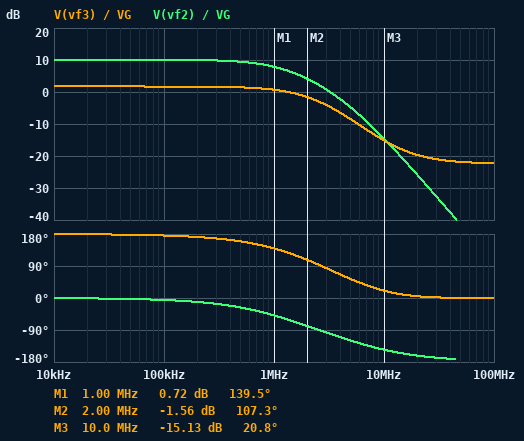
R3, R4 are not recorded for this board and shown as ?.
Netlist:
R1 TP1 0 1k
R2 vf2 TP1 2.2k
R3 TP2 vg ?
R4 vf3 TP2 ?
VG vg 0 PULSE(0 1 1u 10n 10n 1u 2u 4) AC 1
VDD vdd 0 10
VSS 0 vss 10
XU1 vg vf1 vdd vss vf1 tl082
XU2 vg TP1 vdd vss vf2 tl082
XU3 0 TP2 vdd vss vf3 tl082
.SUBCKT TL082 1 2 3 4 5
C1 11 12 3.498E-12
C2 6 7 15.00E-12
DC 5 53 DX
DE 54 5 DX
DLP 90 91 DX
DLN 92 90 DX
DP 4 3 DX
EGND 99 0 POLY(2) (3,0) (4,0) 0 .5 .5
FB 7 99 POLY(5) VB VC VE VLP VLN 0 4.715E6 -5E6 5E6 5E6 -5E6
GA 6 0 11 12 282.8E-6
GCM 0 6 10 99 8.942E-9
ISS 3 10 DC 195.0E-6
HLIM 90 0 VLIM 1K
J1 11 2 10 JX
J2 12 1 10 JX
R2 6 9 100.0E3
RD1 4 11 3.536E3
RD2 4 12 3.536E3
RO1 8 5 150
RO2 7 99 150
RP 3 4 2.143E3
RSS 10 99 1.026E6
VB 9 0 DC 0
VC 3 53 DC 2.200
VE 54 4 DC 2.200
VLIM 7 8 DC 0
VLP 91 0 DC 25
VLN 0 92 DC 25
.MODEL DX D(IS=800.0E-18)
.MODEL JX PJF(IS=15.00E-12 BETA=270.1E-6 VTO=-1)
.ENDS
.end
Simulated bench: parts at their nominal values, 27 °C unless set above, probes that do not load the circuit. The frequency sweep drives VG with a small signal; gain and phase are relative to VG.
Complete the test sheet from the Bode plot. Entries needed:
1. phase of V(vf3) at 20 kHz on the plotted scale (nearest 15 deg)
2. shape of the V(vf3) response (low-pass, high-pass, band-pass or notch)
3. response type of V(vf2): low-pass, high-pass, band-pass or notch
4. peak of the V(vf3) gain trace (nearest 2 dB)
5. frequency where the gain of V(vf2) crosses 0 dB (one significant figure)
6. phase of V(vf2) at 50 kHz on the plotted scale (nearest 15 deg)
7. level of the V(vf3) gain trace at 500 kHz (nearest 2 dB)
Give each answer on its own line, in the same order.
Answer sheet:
180 deg
low-pass
low-pass
2 dB
3 MHz
0 deg
2 dB
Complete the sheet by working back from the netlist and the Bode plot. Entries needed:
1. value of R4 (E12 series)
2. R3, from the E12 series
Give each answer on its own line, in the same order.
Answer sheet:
1 kΩ
820 Ω
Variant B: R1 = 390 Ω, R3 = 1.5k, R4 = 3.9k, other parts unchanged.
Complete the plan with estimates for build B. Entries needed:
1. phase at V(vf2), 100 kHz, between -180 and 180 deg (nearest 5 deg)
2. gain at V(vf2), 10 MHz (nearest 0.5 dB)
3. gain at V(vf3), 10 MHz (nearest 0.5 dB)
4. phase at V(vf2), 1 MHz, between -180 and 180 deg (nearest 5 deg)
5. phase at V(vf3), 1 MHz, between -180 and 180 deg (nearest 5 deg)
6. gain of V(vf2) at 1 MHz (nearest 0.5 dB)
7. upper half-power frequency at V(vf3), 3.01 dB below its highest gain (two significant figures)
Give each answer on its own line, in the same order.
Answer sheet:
-10 deg
-15.0 dB
-16.0 dB
-70 deg
125 deg
10.0 dB
1.1 MHz
